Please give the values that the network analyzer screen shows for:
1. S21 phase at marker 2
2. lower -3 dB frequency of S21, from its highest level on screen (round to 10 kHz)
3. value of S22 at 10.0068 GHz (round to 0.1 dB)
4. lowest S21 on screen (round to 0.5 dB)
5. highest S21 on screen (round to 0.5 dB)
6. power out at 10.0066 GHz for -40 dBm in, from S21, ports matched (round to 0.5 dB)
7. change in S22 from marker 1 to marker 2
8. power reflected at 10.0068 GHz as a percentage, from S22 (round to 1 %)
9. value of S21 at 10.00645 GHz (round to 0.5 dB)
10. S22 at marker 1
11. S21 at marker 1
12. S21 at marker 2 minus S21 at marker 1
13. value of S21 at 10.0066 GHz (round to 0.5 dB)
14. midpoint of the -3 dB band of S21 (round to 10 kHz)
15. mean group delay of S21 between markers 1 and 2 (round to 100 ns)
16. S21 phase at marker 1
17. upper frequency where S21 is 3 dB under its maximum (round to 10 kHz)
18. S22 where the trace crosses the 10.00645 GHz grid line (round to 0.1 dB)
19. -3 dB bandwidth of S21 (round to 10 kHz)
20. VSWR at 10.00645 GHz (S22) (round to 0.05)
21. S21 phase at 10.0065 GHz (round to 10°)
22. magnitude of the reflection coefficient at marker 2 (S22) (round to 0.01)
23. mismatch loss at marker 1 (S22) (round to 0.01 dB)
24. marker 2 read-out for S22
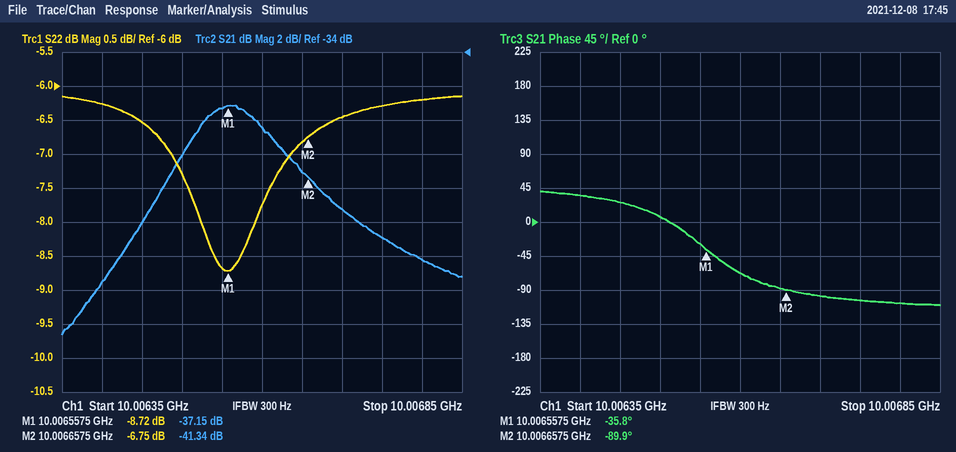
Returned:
-89.9°
10.00650 GHz
-6.2 dB
-50.5 dB
-37.0 dB
-78.5 dBm
1.97 dB
24 %
-44.0 dB
-8.72 dB
-37.15 dB
-4.19 dB
-38.5 dB
10.00657 GHz
1.5 µs
-35.8°
10.00663 GHz
-6.5 dB
130 kHz
2.80
10°
0.46
0.63 dB
-6.75 dB
